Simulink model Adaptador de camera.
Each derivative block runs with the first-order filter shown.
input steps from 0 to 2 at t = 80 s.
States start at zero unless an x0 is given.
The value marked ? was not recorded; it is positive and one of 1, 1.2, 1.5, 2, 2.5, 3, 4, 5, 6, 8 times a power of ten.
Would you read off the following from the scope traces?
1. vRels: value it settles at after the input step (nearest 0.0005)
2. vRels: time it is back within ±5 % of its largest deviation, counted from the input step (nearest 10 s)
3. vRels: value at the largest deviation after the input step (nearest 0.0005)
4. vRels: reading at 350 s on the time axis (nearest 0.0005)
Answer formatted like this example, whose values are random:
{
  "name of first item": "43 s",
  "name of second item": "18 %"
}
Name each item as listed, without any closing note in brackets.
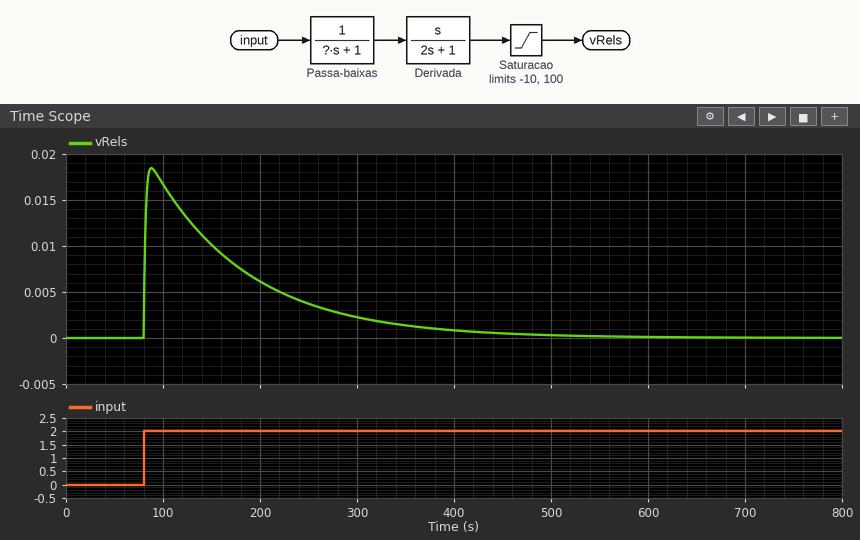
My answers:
{
  "vRels: value it settles at after the input step": "0.0000",
  "vRels: time it is back within ±5 % of its largest deviation, counted from the input step": "310 s",
  "vRels: value at the largest deviation after the input step": "0.0185",
  "vRels: reading at 350 s on the time axis": "0.0015"
}
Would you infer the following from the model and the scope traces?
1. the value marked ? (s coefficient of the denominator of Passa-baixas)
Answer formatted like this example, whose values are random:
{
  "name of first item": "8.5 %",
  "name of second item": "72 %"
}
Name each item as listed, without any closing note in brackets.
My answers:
{
  "the value marked ?": "100"
}
